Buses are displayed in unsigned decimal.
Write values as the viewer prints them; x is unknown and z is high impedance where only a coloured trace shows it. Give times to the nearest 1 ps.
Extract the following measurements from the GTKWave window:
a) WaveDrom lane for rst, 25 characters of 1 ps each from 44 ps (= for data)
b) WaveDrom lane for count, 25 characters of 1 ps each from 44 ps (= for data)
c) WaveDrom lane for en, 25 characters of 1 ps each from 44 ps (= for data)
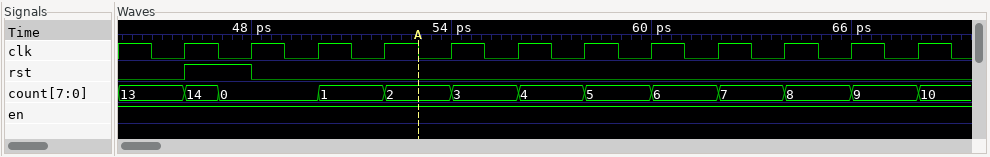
{name: 'rst', wave: '0.1.0....................'}
{name: 'count', wave: '=.==..=.=.=.=.=.=.=.=.=.=', data: '13 14 0 1 2 3 4 5 6 7 8 9 10'}
{name: 'en', wave: '1........................'}
